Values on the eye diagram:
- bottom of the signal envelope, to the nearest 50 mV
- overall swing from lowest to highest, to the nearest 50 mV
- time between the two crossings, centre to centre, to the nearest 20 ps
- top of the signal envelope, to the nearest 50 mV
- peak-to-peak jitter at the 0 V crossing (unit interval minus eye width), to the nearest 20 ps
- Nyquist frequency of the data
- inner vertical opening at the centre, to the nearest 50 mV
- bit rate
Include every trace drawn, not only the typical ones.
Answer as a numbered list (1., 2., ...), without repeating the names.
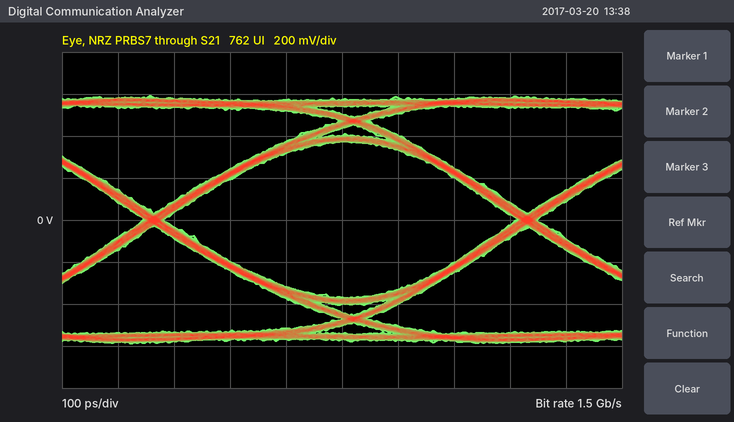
1. -600 mV
2. 1.20 V
3. 660 ps
4. 600 mV
5. 40 ps
6. 750 MHz
7. 750 mV
8. 1.5 Gb/s
